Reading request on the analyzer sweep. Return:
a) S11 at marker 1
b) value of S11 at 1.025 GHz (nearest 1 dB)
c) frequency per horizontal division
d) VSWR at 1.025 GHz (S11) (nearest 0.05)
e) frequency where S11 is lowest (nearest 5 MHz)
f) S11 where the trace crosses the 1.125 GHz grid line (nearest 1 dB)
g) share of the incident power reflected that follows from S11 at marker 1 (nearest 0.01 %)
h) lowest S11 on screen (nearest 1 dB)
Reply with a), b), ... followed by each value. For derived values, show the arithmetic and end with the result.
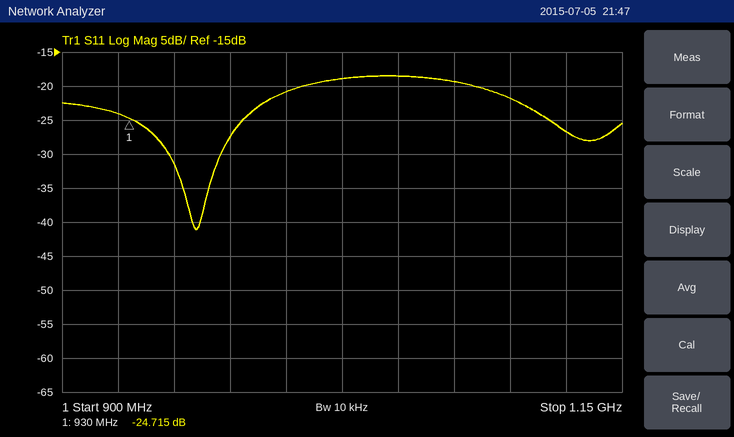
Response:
a) -24.715 dB
b) -19 dB
c) 25 MHz
d) |Γ| = 10^(-19/20) = 0.1122; VSWR = (1 + 0.1122)/(1 − 0.1122) ≈ 1.25
e) 960 MHz
f) -27 dB
g) 10^(-24.715/10) ≈ 0.34 %
h) -41 dB
